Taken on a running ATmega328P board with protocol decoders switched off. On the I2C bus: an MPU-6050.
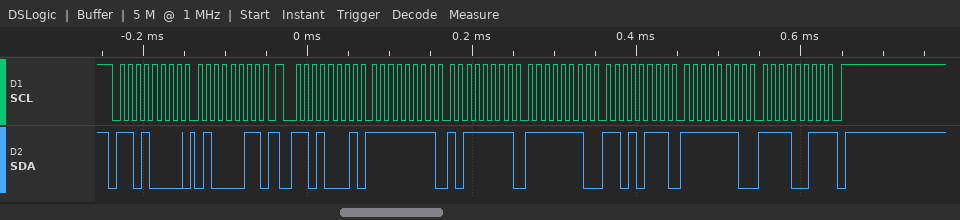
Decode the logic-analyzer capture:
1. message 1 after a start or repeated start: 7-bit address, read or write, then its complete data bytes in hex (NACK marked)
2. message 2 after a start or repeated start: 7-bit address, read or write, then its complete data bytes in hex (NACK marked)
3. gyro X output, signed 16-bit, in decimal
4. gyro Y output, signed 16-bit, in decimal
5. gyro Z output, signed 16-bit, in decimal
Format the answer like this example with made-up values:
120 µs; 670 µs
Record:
0x68 write: 43; 0x68 read: FF BF FE D7 FE F3 NACK; -65; -297; -269
